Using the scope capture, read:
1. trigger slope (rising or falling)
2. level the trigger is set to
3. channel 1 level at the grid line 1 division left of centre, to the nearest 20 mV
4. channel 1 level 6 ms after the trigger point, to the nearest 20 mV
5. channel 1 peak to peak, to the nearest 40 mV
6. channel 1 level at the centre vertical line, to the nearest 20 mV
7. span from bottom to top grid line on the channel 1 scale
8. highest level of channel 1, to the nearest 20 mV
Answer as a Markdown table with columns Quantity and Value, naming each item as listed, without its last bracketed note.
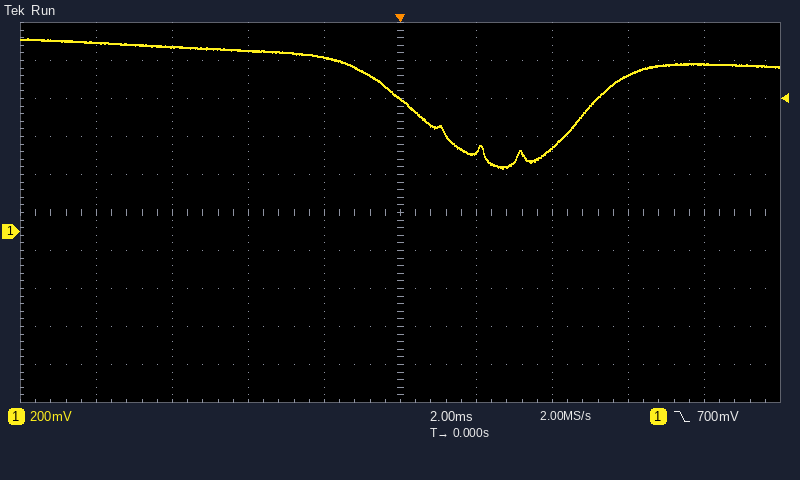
| Quantity | Value |
|---|---|
| trigger slope | falling |
| level the trigger is set to | 700 mV |
| channel 1 level at the grid line 1 division left of centre, to the nearest 20 mV | 920 mV |
| channel 1 level 6 ms after the trigger point, to the nearest 20 mV | 820 mV |
| channel 1 peak to peak, to the nearest 40 mV | 680 mV |
| channel 1 level at the centre vertical line, to the nearest 20 mV | 700 mV |
| span from bottom to top grid line on the channel 1 scale | 2 V |
| highest level of channel 1, to the nearest 20 mV | 1.02 V |
